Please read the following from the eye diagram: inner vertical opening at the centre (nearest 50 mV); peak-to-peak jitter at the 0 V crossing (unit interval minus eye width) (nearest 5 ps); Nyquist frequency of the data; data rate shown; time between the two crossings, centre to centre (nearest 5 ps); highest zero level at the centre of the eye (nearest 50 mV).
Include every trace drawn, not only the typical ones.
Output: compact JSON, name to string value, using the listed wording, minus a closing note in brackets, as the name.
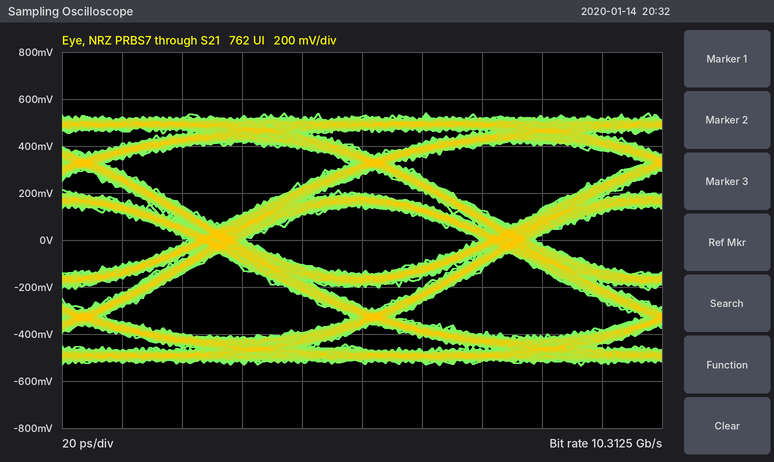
{"inner vertical opening at the centre": "300 mV", "peak-to-peak jitter at the 0 V crossing (unit interval minus eye width)": "20 ps", "Nyquist frequency of the data": "5.15625 GHz", "data rate shown": "10.3125 Gb/s", "time between the two crossings, centre to centre": "95 ps", "highest zero level at the centre of the eye": "-150 mV"}
